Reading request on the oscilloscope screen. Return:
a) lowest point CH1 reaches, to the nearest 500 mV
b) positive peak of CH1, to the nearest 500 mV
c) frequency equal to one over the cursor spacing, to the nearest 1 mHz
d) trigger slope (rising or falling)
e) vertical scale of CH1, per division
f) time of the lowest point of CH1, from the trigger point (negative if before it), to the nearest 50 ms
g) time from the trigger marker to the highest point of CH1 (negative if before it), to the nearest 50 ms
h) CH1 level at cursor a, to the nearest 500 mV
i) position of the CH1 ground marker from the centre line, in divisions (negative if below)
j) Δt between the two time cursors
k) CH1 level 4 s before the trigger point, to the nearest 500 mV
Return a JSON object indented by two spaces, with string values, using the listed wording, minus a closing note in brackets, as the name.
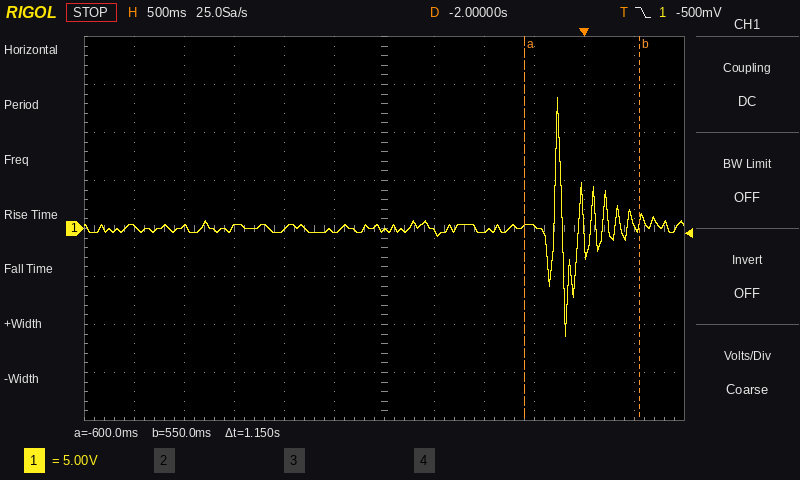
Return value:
{
  "lowest point CH1 reaches, to the nearest 500 mV": "-11.0 V",
  "positive peak of CH1, to the nearest 500 mV": "13.5 V",
  "frequency equal to one over the cursor spacing, to the nearest 1 mHz": "870 mHz",
  "trigger slope": "falling",
  "vertical scale of CH1, per division": "5 V",
  "time of the lowest point of CH1, from the trigger point (negative if before it), to the nearest 50 ms": "-200 ms",
  "time from the trigger marker to the highest point of CH1 (negative if before it), to the nearest 50 ms": "-250 ms",
  "CH1 level at cursor a, to the nearest 500 mV": "0.0 V",
  "position of the CH1 ground marker from the centre line, in divisions": "0.0 div",
  "Δt between the two time cursors": "1.15 s",
  "CH1 level 4 s before the trigger point, to the nearest 500 mV": "0.0 V"
}
